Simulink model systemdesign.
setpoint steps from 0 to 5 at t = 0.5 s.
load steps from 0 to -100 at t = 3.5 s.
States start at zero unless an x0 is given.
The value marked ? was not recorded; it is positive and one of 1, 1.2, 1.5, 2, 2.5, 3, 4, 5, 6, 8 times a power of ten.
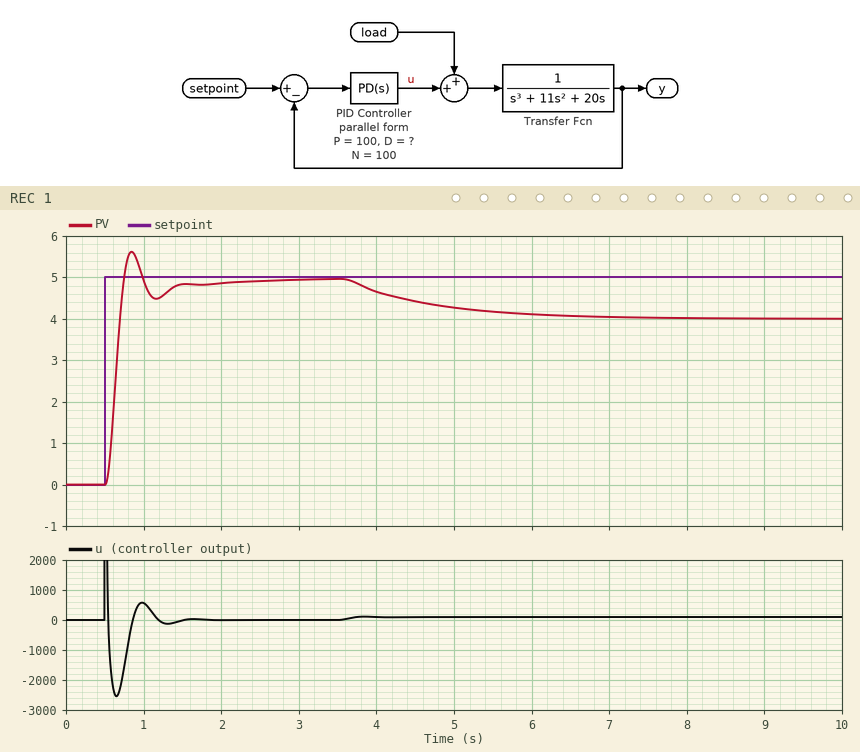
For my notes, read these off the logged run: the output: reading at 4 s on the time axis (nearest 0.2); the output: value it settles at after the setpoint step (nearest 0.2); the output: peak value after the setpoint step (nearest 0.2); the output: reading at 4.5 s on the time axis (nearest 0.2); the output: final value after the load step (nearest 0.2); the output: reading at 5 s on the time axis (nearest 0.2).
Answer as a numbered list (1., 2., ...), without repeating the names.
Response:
1. 4.6
2. 5.0
3. 5.6
4. 4.4
5. 4.0
6. 4.2
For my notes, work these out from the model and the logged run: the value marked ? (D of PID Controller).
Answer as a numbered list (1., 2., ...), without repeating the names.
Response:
1. 100
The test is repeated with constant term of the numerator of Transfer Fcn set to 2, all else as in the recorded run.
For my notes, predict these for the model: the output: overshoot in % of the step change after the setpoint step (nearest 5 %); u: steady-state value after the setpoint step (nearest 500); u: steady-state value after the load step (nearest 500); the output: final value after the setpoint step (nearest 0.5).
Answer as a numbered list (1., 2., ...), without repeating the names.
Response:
1. 35 %
2. 0
3. 0
4. 5.0
